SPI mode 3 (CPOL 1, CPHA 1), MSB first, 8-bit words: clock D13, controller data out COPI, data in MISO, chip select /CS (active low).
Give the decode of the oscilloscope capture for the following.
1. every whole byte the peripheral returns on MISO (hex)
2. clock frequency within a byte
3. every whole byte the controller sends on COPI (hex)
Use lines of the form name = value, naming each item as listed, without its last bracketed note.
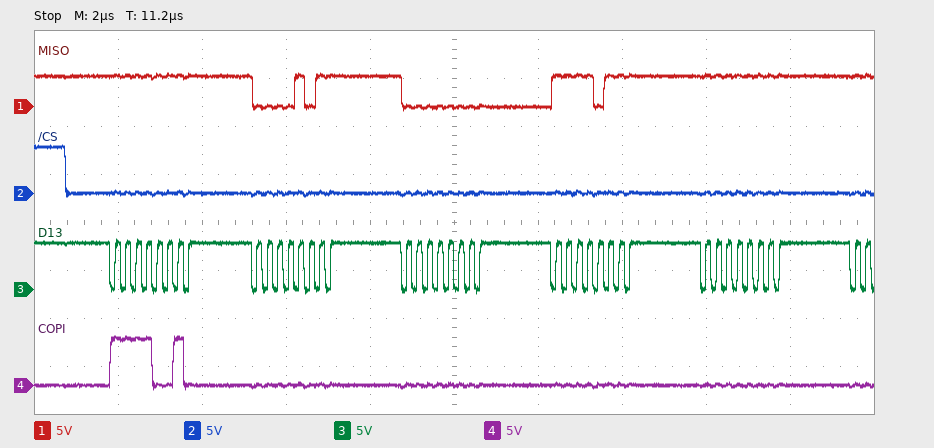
every whole byte the peripheral returns on MISO = FF 0B 00 F7 FF
clock frequency within a byte = 4 MHz
every whole byte the controller sends on COPI = F2 00 00 00 00
